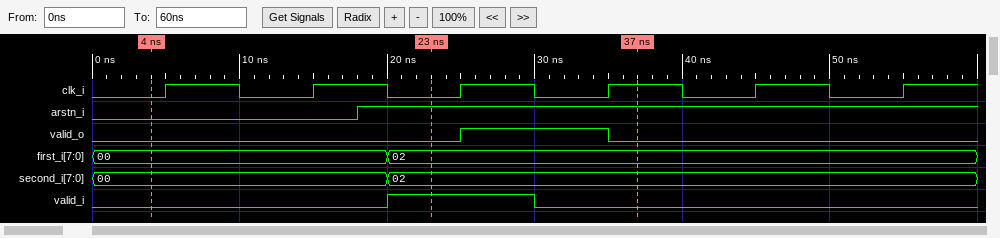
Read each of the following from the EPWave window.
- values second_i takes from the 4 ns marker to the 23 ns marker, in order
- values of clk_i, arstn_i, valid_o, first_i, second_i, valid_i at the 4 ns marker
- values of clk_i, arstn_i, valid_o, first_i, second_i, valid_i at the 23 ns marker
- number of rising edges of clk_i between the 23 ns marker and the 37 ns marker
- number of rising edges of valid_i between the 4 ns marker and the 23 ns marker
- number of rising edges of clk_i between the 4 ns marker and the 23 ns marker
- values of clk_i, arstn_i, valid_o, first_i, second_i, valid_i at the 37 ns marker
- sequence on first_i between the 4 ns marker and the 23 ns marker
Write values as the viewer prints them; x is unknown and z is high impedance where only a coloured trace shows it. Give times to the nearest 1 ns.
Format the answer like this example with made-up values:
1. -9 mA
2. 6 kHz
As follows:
1. 00, 02
2. clk_i=0, arstn_i=0, valid_o=0, first_i=00, second_i=00, valid_i=0
3. clk_i=0, arstn_i=1, valid_o=0, first_i=02, second_i=02, valid_i=1
4. 2
5. 1
6. 2
7. clk_i=1, arstn_i=1, valid_o=0, first_i=02, second_i=02, valid_i=0
8. 00, 02
